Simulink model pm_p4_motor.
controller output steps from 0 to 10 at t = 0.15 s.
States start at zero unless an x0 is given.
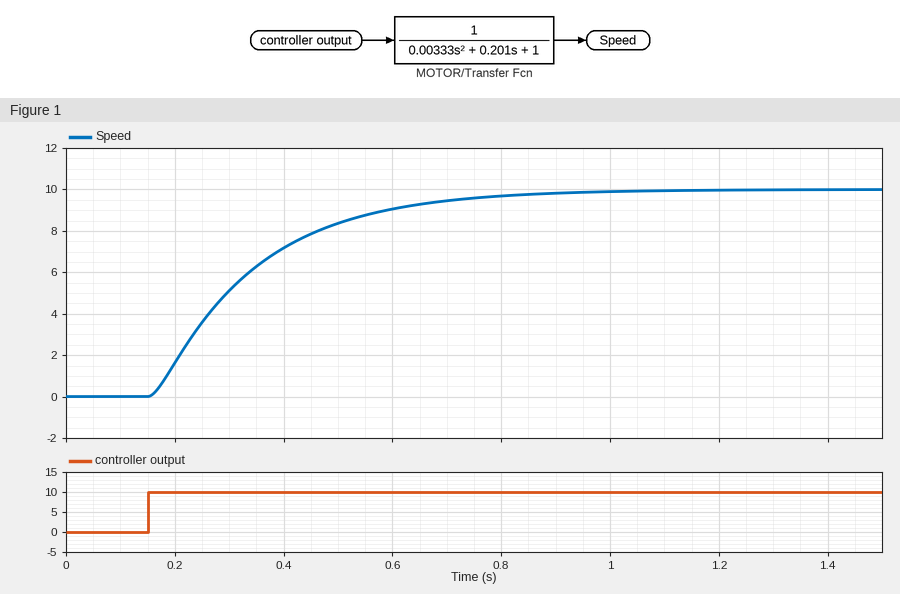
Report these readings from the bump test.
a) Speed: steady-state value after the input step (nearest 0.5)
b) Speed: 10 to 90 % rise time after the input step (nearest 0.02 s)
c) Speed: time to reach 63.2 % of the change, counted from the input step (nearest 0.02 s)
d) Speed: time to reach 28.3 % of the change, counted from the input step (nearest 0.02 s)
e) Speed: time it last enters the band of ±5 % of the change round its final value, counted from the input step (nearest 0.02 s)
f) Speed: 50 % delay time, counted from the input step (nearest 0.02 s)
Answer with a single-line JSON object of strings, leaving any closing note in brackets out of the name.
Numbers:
{"Speed: steady-state value after the input step": "10.0", "Speed: 10 to 90 % rise time after the input step": "0.40 s", "Speed: time to reach 63.2 % of the change, counted from the input step": "0.20 s", "Speed: time to reach 28.3 % of the change, counted from the input step": "0.08 s", "Speed: time it last enters the band of ±5 % of the change round its final value, counted from the input step": "0.56 s", "Speed: 50 % delay time, counted from the input step": "0.14 s"}
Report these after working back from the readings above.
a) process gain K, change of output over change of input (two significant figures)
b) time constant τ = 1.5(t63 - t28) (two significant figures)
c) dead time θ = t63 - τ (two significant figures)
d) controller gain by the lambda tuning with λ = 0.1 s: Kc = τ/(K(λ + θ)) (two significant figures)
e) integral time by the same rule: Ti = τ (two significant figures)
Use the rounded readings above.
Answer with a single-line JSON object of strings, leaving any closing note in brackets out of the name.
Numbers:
{"process gain K, change of output over change of input": "1.0", "time constant τ = 1.5(t63 - t28)": "0.18 s", "dead time θ = t63 - τ": "0.020 s", "controller gain by the lambda tuning with λ = 0.1 s: Kc = τ/(K(λ + θ))": "1.5", "integral time by the same rule: Ti = τ": "0.18 s"}
